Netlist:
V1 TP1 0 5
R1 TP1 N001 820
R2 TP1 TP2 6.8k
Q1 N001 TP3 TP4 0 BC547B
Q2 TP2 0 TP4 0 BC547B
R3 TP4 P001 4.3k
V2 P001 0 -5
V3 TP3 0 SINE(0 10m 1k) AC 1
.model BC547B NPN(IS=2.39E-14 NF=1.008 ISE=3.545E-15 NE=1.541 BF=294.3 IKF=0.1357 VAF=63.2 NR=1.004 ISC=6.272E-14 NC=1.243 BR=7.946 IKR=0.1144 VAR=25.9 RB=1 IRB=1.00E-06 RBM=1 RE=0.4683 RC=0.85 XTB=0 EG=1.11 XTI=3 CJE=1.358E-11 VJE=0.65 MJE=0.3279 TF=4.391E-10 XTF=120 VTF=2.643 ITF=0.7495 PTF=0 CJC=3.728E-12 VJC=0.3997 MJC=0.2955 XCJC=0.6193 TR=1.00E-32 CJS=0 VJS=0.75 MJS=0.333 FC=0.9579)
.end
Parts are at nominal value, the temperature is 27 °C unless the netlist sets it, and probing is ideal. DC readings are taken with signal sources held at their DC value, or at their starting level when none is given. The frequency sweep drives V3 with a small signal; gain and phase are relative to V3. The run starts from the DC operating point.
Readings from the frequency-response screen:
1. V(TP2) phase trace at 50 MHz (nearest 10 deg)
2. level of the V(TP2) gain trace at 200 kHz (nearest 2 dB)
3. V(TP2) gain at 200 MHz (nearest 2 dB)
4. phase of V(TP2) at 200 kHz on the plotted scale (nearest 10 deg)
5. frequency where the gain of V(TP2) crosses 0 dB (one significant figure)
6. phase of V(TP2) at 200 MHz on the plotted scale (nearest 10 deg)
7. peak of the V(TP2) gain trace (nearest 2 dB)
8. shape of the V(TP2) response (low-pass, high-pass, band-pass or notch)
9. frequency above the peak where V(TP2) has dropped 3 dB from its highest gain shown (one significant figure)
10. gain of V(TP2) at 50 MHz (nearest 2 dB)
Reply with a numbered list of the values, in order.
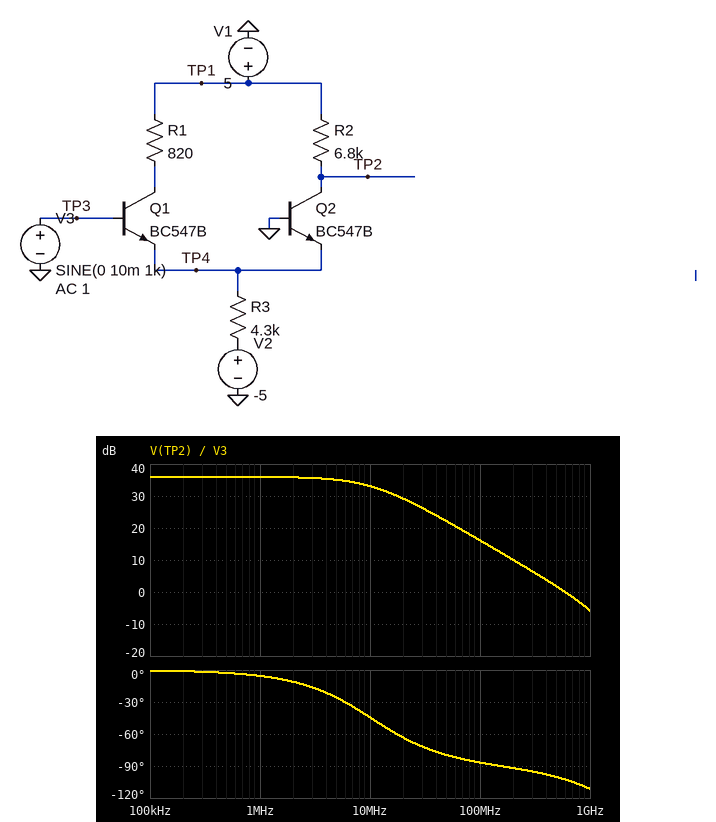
1. -80 deg
2. 36 dB
3. 10 dB
4. 0 deg
5. 600 MHz
6. -90 deg
7. 36 dB
8. low-pass
9. 10 MHz
10. 22 dB
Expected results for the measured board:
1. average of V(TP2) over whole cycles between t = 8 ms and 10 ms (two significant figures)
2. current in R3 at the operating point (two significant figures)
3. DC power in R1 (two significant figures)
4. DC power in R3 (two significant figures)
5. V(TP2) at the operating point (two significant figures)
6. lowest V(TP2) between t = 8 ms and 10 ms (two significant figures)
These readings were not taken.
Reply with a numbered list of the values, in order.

1. 1.6 V
2. 1.0 mA
3. 220 µW
4. 4.5 mW
5. 1.6 V
6. 1.0 V
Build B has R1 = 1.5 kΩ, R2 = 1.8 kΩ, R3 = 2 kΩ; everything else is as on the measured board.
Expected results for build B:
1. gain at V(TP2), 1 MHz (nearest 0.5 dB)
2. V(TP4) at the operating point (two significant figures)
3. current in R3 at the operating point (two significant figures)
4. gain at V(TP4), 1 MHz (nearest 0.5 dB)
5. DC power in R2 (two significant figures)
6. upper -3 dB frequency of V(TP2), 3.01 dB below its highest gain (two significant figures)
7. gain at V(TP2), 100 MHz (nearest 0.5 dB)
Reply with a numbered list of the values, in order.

1. 31.0 dB
2. -640 mV
3. 2.2 mA
4. -6.0 dB
5. 2.1 mW
6. 45 MHz
7. 23.0 dB
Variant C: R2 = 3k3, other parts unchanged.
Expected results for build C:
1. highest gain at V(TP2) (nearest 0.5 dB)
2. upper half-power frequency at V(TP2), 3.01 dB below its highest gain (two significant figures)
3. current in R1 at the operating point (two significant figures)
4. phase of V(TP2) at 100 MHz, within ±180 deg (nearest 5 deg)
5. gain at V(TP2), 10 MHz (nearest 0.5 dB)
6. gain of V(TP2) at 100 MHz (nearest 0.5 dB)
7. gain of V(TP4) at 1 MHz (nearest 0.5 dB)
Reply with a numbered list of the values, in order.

1. 30.0 dB
2. 25 MHz
3. 510 µA
4. -80 deg
5. 29.0 dB
6. 17.5 dB
7. -6.0 dB
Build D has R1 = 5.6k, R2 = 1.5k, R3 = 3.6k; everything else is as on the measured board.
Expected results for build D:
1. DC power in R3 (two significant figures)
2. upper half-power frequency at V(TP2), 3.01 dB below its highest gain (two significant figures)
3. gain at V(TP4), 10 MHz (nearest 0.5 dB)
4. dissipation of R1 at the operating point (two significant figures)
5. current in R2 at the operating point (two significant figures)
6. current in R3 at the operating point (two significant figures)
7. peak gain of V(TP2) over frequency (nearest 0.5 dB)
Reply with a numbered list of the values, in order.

1. 5.3 mW
2. 61 MHz
3. -6.5 dB
4. 2.0 mW
5. 620 µA
6. 1.2 mA
7. 24.5 dB
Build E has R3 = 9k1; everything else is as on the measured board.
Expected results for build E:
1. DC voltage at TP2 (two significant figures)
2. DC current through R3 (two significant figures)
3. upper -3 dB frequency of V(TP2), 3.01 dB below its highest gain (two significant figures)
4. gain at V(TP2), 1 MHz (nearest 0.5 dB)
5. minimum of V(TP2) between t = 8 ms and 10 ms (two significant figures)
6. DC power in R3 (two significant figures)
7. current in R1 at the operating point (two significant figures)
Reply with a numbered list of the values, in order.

1. 3.4 V
2. 480 µA
3. 12 MHz
4. 29.5 dB
5. 3.1 V
6. 2.1 mW
7. 240 µA
